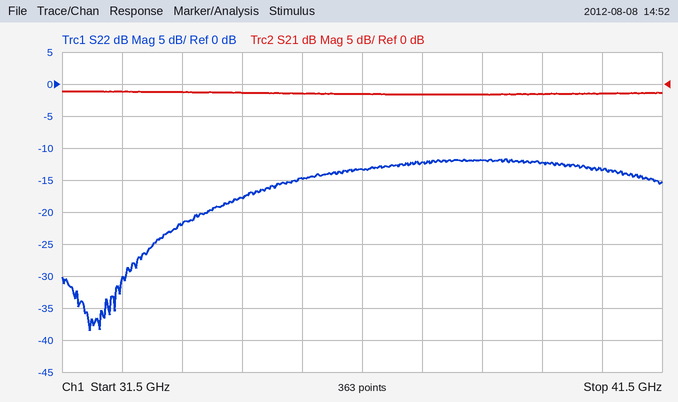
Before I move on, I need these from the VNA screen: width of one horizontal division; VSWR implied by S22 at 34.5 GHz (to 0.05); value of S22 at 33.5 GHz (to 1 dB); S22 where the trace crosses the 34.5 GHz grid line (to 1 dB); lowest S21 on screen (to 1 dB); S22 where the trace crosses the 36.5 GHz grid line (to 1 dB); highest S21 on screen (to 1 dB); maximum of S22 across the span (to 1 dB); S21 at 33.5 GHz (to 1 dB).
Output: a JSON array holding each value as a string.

["1 GHz", "1.30", "-22 dB", "-18 dB", "-2 dB", "-13 dB", "-1 dB", "-12 dB", "-1 dB"]
